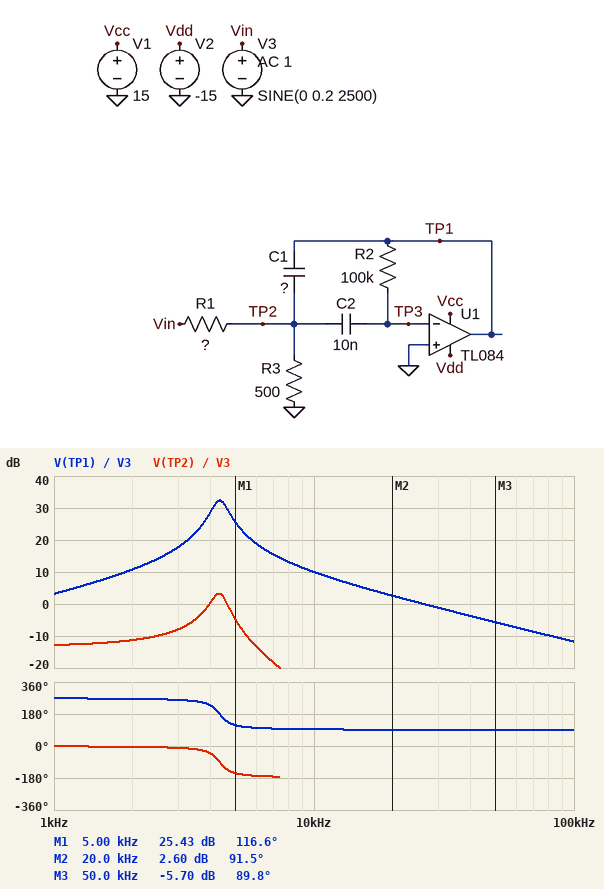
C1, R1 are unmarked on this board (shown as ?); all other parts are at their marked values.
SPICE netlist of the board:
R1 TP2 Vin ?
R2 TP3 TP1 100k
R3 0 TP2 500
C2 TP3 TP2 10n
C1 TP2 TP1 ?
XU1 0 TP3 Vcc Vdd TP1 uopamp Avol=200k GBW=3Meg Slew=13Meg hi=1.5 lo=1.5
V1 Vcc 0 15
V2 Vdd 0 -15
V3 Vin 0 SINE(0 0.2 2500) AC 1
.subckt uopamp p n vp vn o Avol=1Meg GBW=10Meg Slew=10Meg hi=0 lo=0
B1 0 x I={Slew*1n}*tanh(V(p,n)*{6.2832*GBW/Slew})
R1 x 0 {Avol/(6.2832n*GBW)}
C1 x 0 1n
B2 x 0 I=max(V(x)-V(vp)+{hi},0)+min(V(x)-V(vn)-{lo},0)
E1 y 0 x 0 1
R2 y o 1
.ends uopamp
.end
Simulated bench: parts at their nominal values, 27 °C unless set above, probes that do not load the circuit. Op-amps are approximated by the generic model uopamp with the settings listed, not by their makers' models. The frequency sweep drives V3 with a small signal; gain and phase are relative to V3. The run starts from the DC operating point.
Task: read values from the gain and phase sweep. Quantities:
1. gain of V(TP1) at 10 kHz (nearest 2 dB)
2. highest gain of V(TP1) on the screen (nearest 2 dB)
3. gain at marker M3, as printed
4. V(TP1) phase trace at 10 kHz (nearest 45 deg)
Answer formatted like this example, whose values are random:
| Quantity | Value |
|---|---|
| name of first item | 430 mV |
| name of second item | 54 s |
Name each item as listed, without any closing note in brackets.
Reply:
| Quantity | Value |
|---|---|
| gain of V(TP1) at 10 kHz | 10 dB |
| highest gain of V(TP1) on the screen | 32 dB |
| gain at marker M3, as printed | -5.70 dB |
| V(TP1) phase trace at 10 kHz | 90 deg |
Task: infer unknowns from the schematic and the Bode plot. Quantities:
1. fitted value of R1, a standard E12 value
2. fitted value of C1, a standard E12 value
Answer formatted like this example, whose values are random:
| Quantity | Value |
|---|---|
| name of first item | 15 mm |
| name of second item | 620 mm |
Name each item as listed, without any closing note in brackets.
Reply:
| Quantity | Value |
|---|---|
| fitted value of R1, a standard E12 value | 1.8 kΩ |
| fitted value of C1, a standard E12 value | 3.3 nF |
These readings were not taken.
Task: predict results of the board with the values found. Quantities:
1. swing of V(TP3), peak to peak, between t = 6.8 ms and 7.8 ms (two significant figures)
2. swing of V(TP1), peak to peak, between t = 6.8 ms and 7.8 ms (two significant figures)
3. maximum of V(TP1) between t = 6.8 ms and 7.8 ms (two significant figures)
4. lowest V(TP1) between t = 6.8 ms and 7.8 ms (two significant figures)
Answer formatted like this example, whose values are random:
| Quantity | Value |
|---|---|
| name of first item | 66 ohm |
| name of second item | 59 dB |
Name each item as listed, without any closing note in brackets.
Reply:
| Quantity | Value |
|---|---|
| swing of V(TP3), peak to peak, between t = 6.8 ms and 7.8 ms | 1.7 mV |
| swing of V(TP1), peak to peak, between t = 6.8 ms and 7.8 ms | 2.0 V |
| maximum of V(TP1) between t = 6.8 ms and 7.8 ms | 1.0 V |
| lowest V(TP1) between t = 6.8 ms and 7.8 ms | -1.0 V |
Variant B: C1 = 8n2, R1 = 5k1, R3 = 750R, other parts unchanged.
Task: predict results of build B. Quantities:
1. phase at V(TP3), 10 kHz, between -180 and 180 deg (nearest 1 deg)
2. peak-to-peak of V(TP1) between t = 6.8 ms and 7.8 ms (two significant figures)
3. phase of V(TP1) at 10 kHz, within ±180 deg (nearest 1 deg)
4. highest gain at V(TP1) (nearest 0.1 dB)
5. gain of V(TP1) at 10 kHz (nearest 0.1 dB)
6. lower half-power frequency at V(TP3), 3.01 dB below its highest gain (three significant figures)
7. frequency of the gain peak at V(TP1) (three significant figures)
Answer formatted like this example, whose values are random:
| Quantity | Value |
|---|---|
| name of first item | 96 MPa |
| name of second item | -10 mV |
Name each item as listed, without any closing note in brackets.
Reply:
| Quantity | Value |
|---|---|
| phase at V(TP3), 10 kHz, between -180 and 180 deg | 2 deg |
| peak-to-peak of V(TP1) between t = 6.8 ms and 7.8 ms | 2.1 V |
| phase of V(TP1) at 10 kHz, within ±180 deg | 92 deg |
| highest gain at V(TP1) | 20.6 dB |
| gain of V(TP1) at 10 kHz | -8.1 dB |
| lower half-power frequency at V(TP3), 3.01 dB below its highest gain | 2.02 kHz |
| frequency of the gain peak at V(TP1) | 2.16 kHz |
